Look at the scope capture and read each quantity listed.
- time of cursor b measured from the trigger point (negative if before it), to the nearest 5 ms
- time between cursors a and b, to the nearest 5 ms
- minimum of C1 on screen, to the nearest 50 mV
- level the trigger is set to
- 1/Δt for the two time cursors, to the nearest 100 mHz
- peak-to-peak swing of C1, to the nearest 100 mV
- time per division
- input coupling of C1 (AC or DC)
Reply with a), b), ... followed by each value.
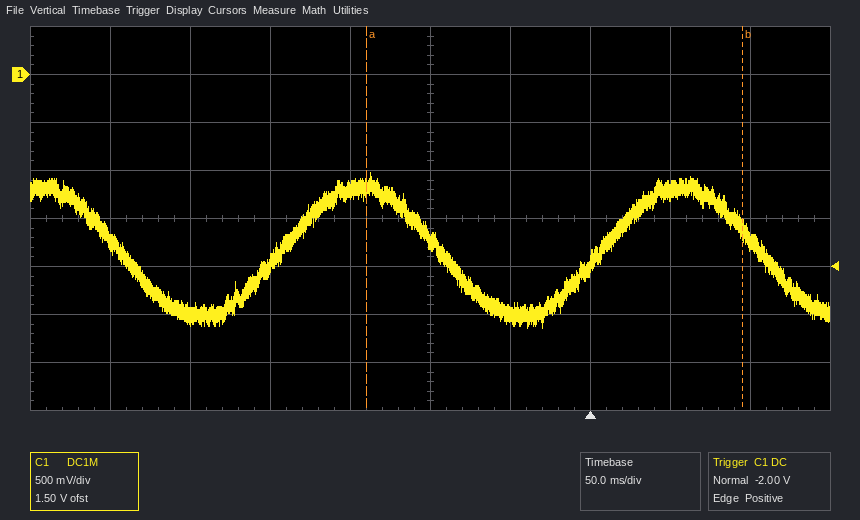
a) +95 ms
b) 235 ms
c) -2.65 V
d) -2.00 V
e) 4.3 Hz
f) 1.60 V
g) 50 ms
h) DC
